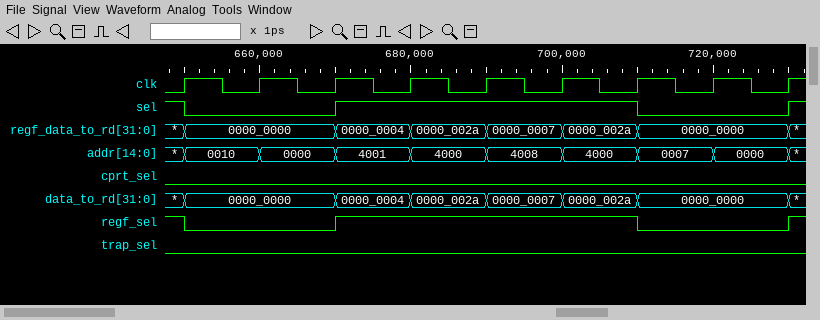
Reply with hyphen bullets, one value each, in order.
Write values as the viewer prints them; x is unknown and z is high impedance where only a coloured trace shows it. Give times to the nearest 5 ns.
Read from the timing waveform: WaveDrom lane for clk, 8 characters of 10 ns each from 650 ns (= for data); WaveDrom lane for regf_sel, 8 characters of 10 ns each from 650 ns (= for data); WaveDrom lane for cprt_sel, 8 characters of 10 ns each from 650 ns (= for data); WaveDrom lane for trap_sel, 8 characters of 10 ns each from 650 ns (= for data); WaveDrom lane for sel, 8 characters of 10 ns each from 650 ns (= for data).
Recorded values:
- {name: 'clk', wave: 'p.......'}
- {name: 'regf_sel', wave: '0.1...0.'}
- {name: 'cprt_sel', wave: '0.......'}
- {name: 'trap_sel', wave: '0.......'}
- {name: 'sel', wave: '0.1...0.'}
